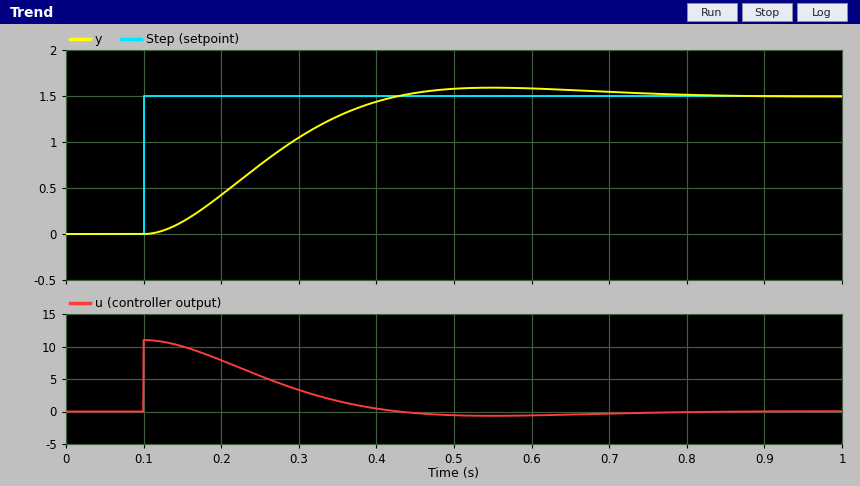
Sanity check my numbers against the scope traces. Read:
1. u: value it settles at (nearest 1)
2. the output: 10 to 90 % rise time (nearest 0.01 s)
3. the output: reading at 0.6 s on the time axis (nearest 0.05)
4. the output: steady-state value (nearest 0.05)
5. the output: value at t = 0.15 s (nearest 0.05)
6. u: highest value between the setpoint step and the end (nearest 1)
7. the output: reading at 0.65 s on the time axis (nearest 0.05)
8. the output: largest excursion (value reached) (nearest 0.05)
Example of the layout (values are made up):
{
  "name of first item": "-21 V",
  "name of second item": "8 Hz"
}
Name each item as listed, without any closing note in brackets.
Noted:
{
  "u: value it settles at": "0",
  "the output: 10 to 90 % rise time": "0.22 s",
  "the output: reading at 0.6 s on the time axis": "1.60",
  "the output: steady-state value": "1.50",
  "the output: value at t = 0.15 s": "0.15",
  "u: highest value between the setpoint step and the end": "11",
  "the output: reading at 0.65 s on the time axis": "1.55",
  "the output: largest excursion (value reached)": "1.60"
}
